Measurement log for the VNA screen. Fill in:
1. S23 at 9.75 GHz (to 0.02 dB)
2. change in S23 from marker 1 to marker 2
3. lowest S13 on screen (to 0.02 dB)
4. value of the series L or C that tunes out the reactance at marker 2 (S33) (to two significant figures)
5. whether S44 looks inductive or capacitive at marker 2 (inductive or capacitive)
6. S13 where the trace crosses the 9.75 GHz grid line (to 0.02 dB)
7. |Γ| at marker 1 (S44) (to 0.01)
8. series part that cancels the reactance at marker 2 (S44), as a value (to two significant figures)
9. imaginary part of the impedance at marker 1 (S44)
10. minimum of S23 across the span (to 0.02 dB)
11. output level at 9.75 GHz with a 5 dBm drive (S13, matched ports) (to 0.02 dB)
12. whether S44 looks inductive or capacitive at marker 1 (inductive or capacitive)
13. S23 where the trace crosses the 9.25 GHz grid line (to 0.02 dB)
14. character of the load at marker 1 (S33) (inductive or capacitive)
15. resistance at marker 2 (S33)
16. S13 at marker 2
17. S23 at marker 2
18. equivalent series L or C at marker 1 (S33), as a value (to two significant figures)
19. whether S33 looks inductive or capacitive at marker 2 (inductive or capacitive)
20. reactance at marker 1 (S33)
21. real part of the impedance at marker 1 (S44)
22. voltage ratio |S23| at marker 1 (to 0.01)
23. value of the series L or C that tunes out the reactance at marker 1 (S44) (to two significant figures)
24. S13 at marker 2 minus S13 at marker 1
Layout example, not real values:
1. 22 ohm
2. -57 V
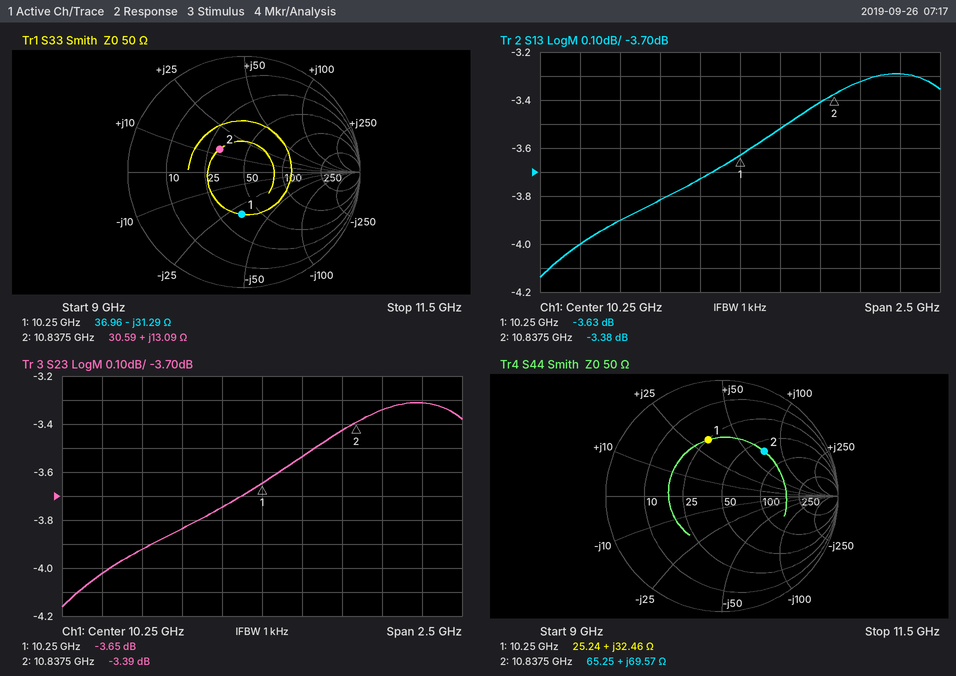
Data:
1. -3.84 dB
2. 0.26 dB
3. -4.14 dB
4. 1.1 pF
5. inductive
6. -3.82 dB
7. 0.50
8. 210 fF
9. +32.46 Ω
10. -4.16 dB
11. 1.18 dBm
12. inductive
13. -4.02 dB
14. capacitive
15. 30.59 Ω
16. -3.38 dB
17. -3.39 dB
18. 500 fF
19. inductive
20. -31.29 Ω
21. 25.24 Ω
22. 0.66
23. 480 fF
24. 0.25 dB
